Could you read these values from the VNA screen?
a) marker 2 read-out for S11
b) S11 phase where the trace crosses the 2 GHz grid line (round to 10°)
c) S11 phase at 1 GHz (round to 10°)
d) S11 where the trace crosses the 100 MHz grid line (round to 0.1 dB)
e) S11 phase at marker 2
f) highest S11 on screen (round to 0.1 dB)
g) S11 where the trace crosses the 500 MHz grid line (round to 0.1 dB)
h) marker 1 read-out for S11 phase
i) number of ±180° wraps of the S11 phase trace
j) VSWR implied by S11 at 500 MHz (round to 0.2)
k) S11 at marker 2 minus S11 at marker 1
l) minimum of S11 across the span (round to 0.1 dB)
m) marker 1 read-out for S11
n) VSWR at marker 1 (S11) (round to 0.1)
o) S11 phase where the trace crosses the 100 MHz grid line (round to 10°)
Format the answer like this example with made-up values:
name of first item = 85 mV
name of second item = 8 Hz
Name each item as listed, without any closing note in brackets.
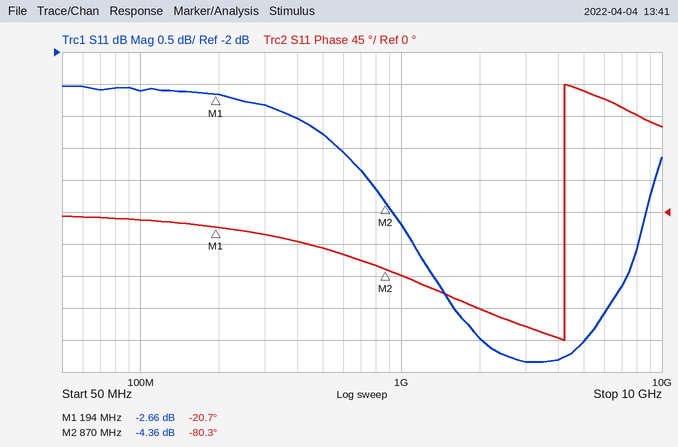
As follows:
marker 2 read-out for S11 = -4.36 dB
S11 phase where the trace crosses the 2 GHz grid line = -140°
S11 phase at 1 GHz = -90°
S11 where the trace crosses the 100 MHz grid line = -2.6 dB
S11 phase at marker 2 = -80.3°
highest S11 on screen = -2.5 dB
S11 where the trace crosses the 500 MHz grid line = -3.3 dB
marker 1 read-out for S11 phase = -20.7°
number of ±180° wraps of the S11 phase trace = 1
VSWR implied by S11 at 500 MHz = 5.4
S11 at marker 2 minus S11 at marker 1 = -1.70 dB
minimum of S11 across the span = -6.8 dB
marker 1 read-out for S11 = -2.66 dB
VSWR at marker 1 (S11) = 6.6
S11 phase where the trace crosses the 100 MHz grid line = -10°
